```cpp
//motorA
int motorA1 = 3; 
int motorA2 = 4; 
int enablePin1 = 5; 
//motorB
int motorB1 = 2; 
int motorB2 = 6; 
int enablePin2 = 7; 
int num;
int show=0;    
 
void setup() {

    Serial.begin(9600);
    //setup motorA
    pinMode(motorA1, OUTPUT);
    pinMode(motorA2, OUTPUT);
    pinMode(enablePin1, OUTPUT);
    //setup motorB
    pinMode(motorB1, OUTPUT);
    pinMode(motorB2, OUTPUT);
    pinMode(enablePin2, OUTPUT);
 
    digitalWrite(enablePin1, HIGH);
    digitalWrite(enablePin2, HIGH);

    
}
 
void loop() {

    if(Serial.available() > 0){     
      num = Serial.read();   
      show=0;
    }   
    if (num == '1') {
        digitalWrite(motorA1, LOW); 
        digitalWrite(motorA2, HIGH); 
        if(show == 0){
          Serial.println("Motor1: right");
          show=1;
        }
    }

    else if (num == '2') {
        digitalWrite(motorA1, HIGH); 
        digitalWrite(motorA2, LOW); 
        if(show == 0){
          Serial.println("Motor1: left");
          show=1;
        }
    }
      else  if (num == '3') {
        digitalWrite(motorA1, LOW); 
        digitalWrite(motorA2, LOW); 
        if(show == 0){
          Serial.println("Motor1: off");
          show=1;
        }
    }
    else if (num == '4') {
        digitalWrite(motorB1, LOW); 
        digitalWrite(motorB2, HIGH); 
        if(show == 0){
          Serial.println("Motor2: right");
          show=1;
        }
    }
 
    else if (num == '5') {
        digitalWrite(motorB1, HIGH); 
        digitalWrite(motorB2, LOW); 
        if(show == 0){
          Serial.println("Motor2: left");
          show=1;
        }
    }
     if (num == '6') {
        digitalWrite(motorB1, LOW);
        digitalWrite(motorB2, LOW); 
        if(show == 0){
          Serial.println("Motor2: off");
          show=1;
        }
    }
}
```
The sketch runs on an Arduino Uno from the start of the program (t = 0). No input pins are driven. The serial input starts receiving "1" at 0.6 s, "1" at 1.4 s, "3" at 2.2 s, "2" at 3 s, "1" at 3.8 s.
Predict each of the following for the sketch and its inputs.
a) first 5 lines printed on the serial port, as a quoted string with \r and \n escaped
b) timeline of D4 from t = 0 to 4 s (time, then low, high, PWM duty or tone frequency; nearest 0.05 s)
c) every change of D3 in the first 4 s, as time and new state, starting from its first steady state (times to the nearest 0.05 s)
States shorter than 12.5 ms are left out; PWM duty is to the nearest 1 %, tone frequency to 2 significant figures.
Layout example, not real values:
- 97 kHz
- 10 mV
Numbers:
- "Motor1: right\r\nMotor1: right\r\nMotor1: off\r\nMotor1: left\r\nMotor1: right\r\n"
- 0 s low; 0.6 s high; 2.2 s low; 3.8 s high
- 0 s low; 3 s high; 3.8 s low
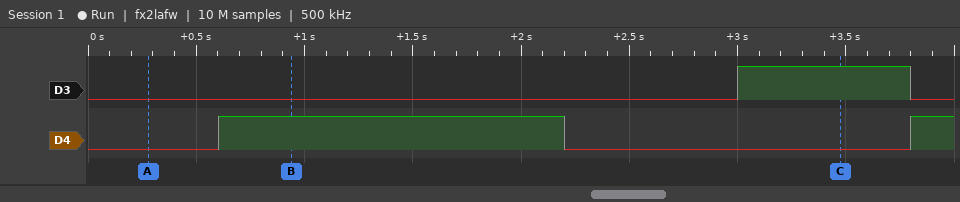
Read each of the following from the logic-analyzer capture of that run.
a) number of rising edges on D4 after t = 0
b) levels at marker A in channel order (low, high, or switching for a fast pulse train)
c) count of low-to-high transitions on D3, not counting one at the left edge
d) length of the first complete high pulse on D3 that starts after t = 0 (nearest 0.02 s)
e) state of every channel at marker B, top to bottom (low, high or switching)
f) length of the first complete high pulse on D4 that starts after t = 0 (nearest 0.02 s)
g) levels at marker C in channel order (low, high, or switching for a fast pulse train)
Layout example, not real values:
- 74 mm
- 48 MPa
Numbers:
- 2
- D3 low, D4 low
- 1
- 0.80 s
- D3 low, D4 high
- 1.60 s
- D3 high, D4 low
